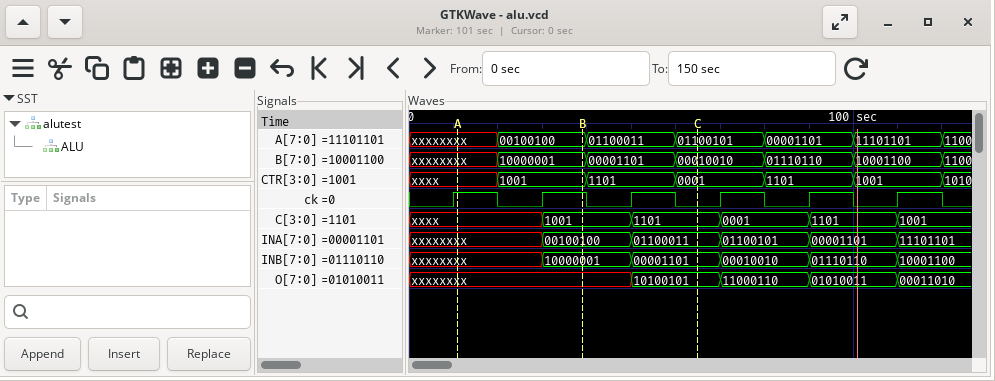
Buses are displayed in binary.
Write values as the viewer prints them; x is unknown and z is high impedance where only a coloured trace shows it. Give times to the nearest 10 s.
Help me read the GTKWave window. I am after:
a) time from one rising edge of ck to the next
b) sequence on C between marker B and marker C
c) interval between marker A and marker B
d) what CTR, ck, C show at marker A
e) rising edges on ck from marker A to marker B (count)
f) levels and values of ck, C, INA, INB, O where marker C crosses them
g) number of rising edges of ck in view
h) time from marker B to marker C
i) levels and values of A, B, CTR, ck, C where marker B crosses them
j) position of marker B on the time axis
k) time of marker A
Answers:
20 s
1001, 1101
30 s
CTR=xxxx, ck=1, C=xxxx
1
ck=0, C=1101, INA=01100011, INB=00001101, O=10100101
6
30 s
A=00100100, B=10000001, CTR=1001, ck=1, C=1001
40 s
10 s
